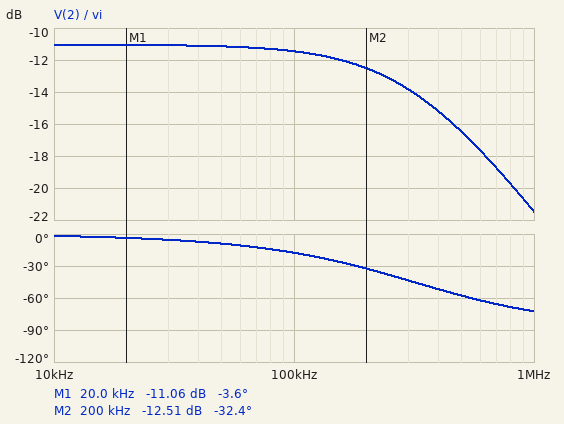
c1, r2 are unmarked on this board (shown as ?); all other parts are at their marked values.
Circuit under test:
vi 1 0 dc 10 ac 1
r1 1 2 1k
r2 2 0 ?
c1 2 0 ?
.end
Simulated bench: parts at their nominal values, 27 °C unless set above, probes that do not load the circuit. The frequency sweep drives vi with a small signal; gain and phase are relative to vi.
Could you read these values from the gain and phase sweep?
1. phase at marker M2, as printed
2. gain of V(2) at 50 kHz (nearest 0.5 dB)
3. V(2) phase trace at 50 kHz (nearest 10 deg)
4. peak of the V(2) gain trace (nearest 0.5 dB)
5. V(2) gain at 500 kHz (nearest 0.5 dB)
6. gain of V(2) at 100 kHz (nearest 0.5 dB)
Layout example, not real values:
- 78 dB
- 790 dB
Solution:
- -32.4 deg
- -11.0 dB
- -10 deg
- -11.0 dB
- -16.5 dB
- -11.5 dB
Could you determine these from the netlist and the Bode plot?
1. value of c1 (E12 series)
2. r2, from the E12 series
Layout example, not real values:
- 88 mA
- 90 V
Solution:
- 1.8 nF
- 390 Ω
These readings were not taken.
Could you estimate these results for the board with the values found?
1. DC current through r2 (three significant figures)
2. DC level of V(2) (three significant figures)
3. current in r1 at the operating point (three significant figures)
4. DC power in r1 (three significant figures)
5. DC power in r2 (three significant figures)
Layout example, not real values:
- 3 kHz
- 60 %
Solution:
- 7.19 mA
- 2.81 V
- 7.19 mA
- 51.8 mW
- 20.2 mW
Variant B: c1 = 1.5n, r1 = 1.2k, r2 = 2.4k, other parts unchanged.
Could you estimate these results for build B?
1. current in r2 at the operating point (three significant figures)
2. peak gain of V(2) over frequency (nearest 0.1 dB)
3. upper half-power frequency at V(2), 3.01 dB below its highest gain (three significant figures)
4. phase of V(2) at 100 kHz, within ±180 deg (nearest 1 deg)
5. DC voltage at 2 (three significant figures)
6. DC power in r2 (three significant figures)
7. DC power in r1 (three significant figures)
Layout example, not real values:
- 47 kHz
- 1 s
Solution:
- 2.78 mA
- -3.5 dB
- 133 kHz
- -37 deg
- 6.67 V
- 18.5 mW
- 9.26 mW
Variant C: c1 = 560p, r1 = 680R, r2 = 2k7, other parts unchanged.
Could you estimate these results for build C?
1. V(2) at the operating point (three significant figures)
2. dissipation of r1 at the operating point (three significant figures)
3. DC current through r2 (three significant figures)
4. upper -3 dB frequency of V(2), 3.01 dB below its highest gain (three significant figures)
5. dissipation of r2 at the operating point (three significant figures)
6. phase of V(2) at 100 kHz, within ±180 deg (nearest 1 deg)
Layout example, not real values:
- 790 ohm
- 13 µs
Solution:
- 7.99 V
- 5.95 mW
- 2.96 mA
- 523 kHz
- 23.6 mW
- -11 deg
